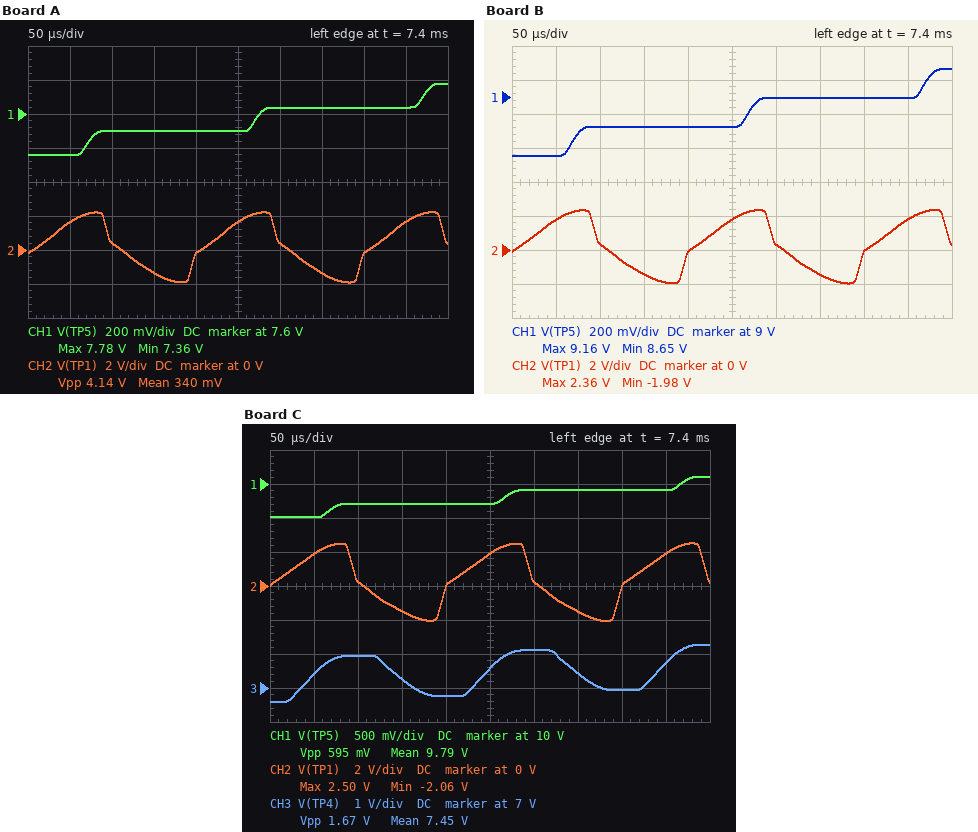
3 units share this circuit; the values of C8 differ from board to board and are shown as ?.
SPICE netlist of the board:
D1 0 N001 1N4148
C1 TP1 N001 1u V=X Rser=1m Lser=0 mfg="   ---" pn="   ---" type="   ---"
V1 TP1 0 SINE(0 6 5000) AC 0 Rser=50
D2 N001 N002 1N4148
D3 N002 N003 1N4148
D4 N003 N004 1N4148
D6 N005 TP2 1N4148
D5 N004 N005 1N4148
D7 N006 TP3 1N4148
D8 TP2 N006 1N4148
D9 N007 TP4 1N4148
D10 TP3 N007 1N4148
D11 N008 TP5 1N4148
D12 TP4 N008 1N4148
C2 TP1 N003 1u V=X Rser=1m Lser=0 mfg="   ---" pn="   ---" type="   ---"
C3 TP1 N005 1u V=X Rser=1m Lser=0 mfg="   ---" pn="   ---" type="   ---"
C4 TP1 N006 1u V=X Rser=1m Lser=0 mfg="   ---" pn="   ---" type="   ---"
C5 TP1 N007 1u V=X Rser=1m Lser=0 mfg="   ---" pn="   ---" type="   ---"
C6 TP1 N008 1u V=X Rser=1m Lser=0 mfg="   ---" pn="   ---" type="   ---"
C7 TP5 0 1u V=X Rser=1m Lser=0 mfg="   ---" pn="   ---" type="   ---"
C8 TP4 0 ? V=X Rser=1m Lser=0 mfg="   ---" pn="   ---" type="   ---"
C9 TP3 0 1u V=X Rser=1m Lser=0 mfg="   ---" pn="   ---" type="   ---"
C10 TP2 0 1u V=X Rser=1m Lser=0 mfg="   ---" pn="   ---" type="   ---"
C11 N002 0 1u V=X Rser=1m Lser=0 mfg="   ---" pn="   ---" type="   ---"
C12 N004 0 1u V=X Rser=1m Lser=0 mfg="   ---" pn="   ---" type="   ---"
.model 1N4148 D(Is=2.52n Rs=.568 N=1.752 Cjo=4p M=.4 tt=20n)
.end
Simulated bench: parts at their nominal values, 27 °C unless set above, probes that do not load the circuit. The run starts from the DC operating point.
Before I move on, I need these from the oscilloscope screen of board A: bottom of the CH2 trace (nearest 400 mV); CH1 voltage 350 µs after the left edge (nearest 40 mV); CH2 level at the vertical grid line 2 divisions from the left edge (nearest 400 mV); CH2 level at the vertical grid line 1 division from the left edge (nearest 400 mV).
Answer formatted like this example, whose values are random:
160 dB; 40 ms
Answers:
-2.0 V; 7.64 V; 400 mV; 1.6 V
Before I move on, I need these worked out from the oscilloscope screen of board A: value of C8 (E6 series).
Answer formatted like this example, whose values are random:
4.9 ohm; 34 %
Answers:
3.3 µF
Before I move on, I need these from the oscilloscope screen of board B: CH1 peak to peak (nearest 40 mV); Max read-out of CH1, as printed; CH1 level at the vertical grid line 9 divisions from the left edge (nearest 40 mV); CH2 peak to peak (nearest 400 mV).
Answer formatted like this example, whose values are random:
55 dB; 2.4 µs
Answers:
520 mV; 9.16 V; 9.00 V; 4.4 V
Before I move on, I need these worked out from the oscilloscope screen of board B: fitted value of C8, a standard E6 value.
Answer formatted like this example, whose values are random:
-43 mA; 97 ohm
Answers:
1.5 µF
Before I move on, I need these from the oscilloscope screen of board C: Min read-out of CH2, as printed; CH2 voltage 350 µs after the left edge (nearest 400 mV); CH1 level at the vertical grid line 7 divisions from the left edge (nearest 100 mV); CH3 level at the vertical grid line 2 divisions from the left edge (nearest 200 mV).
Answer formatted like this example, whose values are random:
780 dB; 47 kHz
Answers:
-2.06 V; -1.6 V; 9.9 V; 8.0 V
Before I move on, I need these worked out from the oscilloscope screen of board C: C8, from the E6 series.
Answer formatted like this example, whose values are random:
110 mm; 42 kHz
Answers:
330 nF
